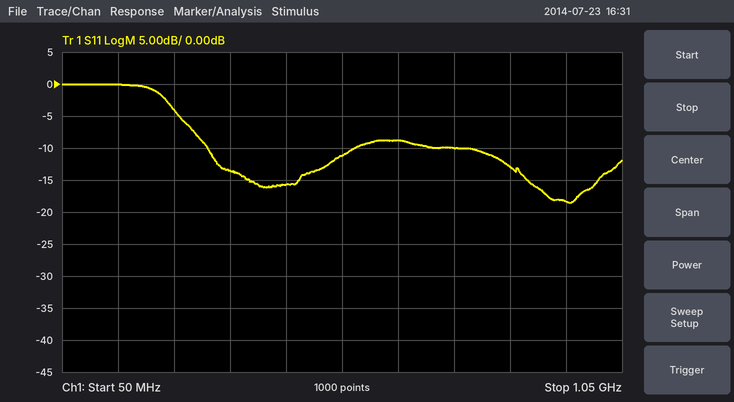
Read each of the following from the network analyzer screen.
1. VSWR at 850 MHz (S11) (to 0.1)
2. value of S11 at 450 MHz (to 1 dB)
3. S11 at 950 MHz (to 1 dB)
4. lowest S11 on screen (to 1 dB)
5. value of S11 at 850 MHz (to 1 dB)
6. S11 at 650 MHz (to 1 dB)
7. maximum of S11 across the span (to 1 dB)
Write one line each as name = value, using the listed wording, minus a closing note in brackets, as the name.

VSWR at 850 MHz (S11) = 1.6
value of S11 at 450 MHz = -16 dB
S11 at 950 MHz = -18 dB
lowest S11 on screen = -19 dB
value of S11 at 850 MHz = -13 dB
S11 at 650 MHz = -9 dB
maximum of S11 across the span = 0 dB
